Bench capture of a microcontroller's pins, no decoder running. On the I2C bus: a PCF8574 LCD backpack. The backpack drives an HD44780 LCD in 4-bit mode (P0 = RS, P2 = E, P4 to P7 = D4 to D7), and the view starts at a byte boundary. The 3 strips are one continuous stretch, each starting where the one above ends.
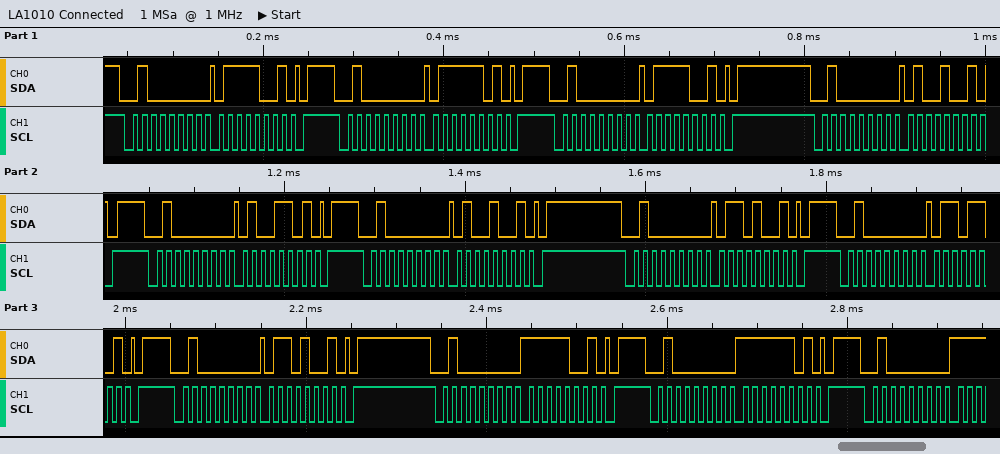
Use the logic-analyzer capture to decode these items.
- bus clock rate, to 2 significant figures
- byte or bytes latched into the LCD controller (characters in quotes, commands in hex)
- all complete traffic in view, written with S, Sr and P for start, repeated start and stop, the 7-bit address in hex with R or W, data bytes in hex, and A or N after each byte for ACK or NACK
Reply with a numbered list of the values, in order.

1. 100 kHz
2. 't'
3. S 20W A 79 A P S 20W A 7D A P S 20W A 79 A P S 20W A 49 A P S 20W A 4D A P S 20W A 49 A P S 20W A 69 A P S 20W A 6D A P S 20W A 69 A P S 20W A F9 A P S 20W A FD A P S 20W A
